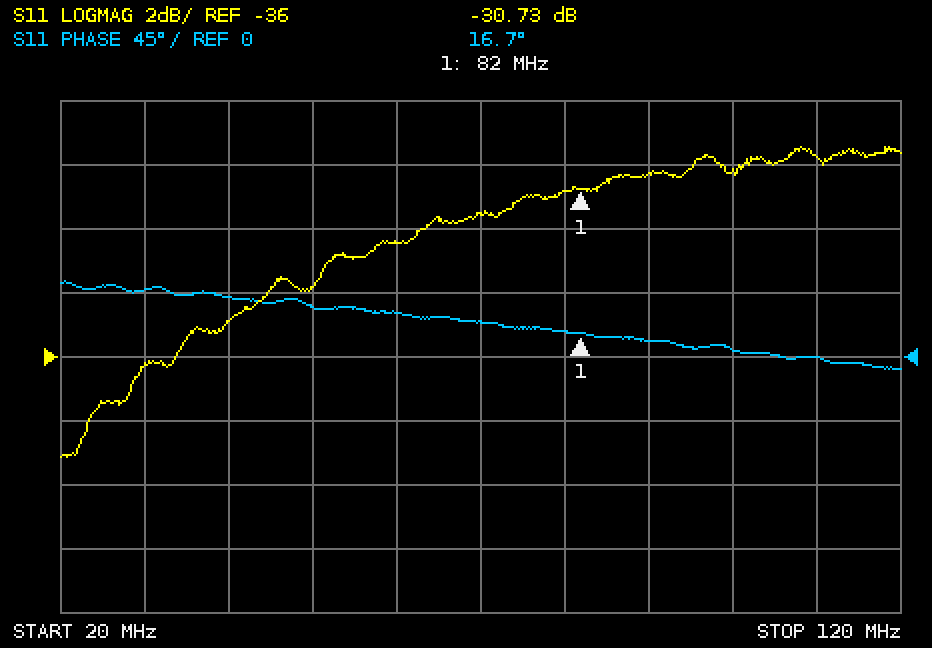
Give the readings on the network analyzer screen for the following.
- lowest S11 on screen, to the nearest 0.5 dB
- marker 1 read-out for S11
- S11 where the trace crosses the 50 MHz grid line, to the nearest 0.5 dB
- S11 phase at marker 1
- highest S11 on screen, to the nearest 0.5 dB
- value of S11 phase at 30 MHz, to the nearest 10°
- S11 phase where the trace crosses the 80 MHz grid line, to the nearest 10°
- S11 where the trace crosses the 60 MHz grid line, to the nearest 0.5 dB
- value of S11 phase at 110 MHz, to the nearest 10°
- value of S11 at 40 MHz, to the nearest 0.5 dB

-39.0 dB
-30.73 dB
-34.0 dB
16.7°
-29.5 dB
50°
20°
-32.5 dB
0°
-35.0 dB
